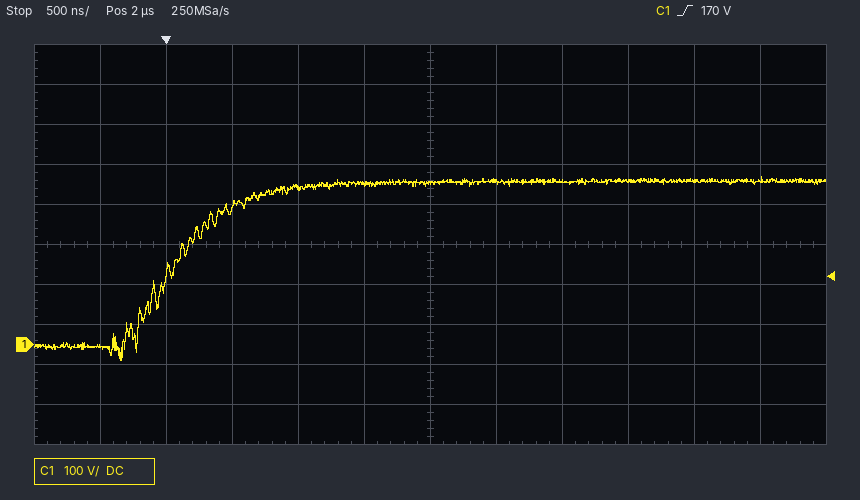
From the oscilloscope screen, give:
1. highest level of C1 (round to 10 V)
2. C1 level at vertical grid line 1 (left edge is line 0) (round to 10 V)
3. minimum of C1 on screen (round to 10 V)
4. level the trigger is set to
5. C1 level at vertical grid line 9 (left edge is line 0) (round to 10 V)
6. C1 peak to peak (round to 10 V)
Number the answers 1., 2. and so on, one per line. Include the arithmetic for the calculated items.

1. 420 V
2. -10 V
3. -40 V
4. 170 V
5. 410 V
6. 420 V − (-40 V) = 460 V
